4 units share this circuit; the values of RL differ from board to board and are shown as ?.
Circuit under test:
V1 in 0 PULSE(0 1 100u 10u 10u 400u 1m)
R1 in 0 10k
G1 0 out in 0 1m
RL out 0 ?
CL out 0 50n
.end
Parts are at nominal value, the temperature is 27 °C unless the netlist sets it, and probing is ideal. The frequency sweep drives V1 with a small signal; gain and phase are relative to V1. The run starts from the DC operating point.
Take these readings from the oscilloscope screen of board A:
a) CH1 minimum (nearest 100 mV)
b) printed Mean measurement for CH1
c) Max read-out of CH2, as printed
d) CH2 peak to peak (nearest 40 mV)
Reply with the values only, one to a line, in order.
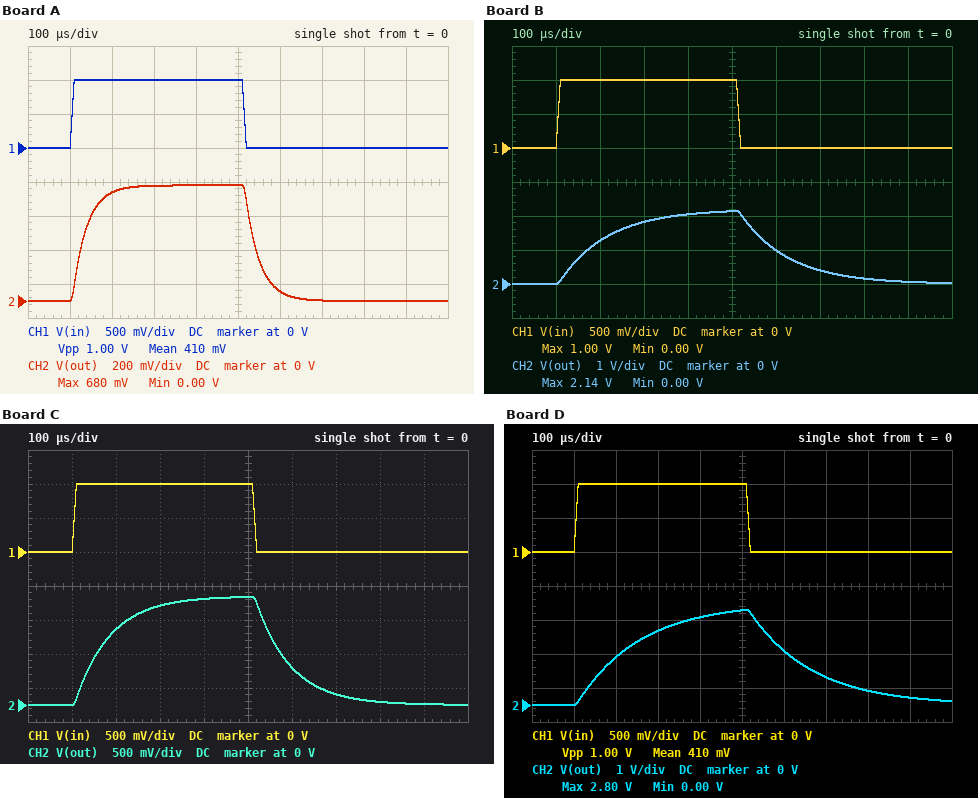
0 V
410 mV
680 mV
680 mV
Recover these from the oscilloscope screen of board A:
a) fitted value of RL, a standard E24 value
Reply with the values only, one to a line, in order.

680 Ω
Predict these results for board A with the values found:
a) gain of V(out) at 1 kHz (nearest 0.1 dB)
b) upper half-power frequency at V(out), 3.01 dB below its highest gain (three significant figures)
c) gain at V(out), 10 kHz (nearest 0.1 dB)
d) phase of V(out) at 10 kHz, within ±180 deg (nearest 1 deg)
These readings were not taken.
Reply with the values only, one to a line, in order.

-3.5 dB
4.68 kHz
-10.8 dB
-65 deg
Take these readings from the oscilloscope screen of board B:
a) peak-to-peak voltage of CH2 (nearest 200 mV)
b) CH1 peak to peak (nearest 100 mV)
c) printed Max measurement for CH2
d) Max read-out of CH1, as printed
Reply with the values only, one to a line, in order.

2.2 V
1.0 V
2.14 V
1.00 V
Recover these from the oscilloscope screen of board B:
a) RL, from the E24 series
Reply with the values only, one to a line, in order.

2.2 kΩ
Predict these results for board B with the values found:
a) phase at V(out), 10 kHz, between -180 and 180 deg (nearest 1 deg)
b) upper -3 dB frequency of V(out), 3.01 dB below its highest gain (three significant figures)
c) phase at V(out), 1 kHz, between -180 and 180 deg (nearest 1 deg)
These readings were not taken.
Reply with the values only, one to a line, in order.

-82 deg
1.45 kHz
-35 deg
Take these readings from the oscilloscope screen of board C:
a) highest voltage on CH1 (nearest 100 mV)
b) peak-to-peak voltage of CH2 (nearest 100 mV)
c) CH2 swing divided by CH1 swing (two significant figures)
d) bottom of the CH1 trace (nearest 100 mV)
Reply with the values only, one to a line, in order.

1.0 V
1.6 V
1.6
0 V
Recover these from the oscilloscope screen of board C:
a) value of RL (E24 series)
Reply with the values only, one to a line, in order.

1.6 kΩ
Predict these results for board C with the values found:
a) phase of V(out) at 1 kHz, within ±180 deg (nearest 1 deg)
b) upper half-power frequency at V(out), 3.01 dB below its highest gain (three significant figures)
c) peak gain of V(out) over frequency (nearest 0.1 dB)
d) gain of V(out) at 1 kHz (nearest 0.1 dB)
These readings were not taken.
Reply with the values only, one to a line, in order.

-27 deg
1.99 kHz
4.1 dB
3.1 dB
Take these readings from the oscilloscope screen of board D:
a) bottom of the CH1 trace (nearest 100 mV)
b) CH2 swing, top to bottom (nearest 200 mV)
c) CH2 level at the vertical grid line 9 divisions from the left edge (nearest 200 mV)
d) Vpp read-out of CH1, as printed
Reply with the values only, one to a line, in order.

0 V
2.8 V
200 mV
1.00 V
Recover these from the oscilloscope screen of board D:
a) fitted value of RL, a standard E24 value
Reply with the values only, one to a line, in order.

3 kΩ
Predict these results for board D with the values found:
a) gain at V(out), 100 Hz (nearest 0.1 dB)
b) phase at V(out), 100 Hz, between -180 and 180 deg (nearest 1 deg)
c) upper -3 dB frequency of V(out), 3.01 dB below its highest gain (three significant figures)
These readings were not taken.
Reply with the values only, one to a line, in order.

9.5 dB
-5 deg
1.06 kHz
